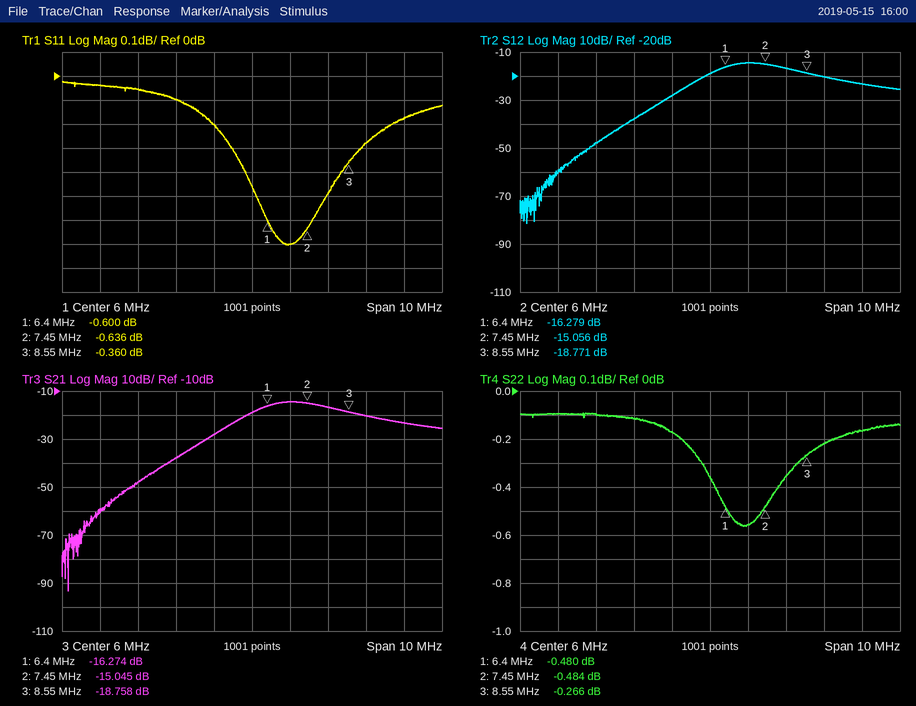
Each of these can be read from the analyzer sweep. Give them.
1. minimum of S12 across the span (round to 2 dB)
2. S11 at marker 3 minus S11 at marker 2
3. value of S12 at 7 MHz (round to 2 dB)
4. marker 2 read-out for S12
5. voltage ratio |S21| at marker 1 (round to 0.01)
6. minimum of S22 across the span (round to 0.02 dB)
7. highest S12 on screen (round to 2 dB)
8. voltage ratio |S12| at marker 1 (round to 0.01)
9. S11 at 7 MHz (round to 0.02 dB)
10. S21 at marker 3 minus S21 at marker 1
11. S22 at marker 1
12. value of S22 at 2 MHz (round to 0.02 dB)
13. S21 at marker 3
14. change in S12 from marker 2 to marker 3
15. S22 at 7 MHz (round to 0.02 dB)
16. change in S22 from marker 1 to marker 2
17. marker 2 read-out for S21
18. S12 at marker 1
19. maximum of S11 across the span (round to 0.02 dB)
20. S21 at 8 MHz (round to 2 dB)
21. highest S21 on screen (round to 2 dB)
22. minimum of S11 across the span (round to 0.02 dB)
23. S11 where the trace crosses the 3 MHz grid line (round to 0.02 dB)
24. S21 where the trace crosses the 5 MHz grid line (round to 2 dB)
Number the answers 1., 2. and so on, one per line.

1. -82 dB
2. 0.276 dB
3. -14 dB
4. -15.056 dB
5. 0.15
6. -0.56 dB
7. -14 dB
8. 0.15
9. -0.70 dB
10. -2.484 dB
11. -0.480 dB
12. -0.10 dB
13. -18.758 dB
14. -3.715 dB
15. -0.56 dB
16. -0.004 dB
17. -15.045 dB
18. -16.279 dB
19. -0.02 dB
20. -16 dB
21. -14 dB
22. -0.70 dB
23. -0.06 dB
24. -28 dB
